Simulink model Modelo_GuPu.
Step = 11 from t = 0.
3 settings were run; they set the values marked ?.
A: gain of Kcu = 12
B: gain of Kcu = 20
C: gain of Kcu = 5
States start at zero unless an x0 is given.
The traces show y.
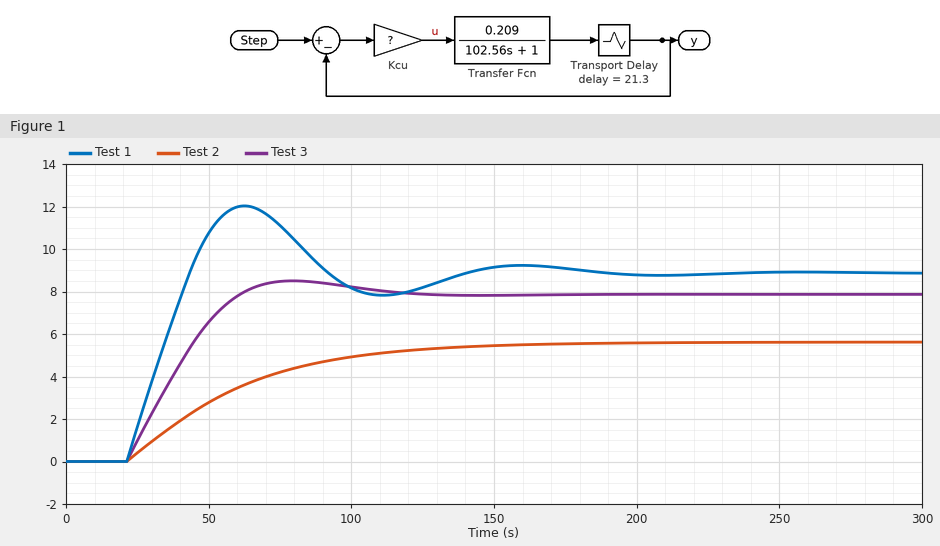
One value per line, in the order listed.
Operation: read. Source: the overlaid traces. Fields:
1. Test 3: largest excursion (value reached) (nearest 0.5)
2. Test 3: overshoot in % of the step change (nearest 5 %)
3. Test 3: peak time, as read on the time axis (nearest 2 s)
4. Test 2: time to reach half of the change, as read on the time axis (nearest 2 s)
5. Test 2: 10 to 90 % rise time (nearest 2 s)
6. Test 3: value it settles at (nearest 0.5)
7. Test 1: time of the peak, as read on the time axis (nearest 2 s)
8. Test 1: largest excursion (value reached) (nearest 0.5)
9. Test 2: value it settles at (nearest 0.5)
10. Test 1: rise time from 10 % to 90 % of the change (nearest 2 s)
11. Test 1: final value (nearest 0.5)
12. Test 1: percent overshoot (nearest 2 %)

8.5
10 %
80 s
50 s
82 s
8.0
62 s
12.0
5.5
18 s
9.0
36 %
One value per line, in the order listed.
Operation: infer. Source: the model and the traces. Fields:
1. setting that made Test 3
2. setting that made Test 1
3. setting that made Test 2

A
B
C
